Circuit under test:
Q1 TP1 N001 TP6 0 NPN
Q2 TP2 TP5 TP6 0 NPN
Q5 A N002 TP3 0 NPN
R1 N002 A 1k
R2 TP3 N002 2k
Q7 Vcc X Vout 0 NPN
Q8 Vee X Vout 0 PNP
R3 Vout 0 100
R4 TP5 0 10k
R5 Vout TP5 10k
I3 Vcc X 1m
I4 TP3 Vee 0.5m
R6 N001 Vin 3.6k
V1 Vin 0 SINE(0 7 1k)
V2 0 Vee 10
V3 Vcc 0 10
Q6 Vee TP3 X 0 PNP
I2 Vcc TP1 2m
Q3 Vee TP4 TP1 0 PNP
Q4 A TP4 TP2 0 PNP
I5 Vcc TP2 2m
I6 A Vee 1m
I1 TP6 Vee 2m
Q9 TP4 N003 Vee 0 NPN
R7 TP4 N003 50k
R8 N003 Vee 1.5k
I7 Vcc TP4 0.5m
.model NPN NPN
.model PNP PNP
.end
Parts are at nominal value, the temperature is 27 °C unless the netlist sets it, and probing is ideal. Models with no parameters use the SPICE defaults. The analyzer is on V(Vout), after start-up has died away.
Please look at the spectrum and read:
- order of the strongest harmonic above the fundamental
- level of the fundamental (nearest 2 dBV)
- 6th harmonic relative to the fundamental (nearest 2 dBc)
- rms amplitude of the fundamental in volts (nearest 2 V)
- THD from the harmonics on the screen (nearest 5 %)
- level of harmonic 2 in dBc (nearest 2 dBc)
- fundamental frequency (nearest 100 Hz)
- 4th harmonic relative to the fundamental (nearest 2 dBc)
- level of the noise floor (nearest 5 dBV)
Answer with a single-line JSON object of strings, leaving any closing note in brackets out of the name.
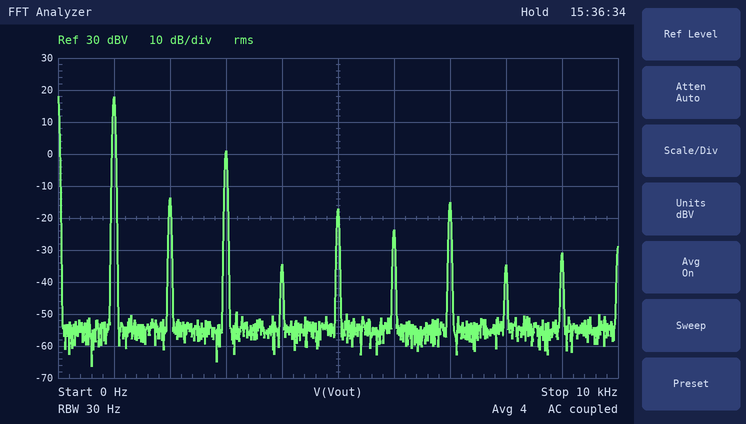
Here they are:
{"order of the strongest harmonic above the fundamental": "3", "level of the fundamental": "18 dBV", "6th harmonic relative to the fundamental": "-42 dBc", "rms amplitude of the fundamental in volts": "8 V", "THD from the harmonics on the screen": "15 %", "level of harmonic 2 in dBc": "-32 dBc", "fundamental frequency": "1.0 kHz", "4th harmonic relative to the fundamental": "-52 dBc", "level of the noise floor": "-55 dBV"}
